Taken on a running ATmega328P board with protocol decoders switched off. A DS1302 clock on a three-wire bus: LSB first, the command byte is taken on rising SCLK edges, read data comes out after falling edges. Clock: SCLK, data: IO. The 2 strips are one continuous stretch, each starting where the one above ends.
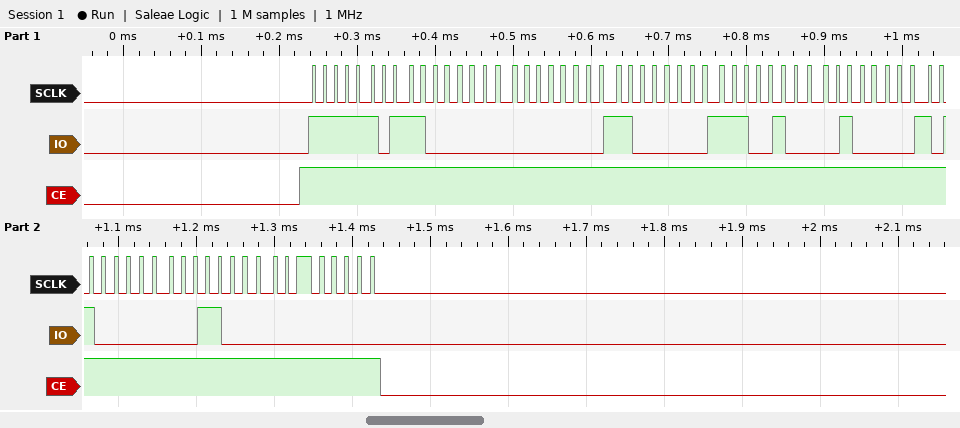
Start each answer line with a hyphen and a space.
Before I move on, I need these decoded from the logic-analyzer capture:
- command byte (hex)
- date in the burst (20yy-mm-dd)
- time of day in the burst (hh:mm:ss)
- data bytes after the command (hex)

- 0xBF
- 2018-04-27
- 03:00:03
- 03 00 03 27 04 05 18 00
